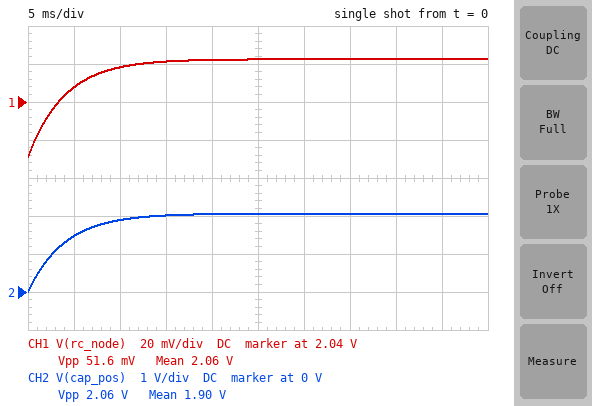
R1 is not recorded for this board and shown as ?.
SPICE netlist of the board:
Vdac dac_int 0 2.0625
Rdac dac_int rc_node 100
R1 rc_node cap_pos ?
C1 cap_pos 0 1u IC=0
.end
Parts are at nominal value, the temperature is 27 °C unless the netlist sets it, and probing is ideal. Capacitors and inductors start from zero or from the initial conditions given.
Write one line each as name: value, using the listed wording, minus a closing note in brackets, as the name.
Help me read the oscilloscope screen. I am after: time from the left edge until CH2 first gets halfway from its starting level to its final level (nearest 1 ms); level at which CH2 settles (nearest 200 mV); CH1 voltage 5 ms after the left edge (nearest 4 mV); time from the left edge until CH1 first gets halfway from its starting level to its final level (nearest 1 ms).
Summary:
time from the left edge until CH2 first gets halfway from its starting level to its final level: 3 ms
level at which CH2 settles: 2.0 V
CH1 voltage 5 ms after the left edge: 2.048 V
time from the left edge until CH1 first gets halfway from its starting level to its final level: 3 ms
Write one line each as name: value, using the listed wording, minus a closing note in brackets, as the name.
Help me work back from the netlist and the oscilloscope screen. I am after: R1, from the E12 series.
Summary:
R1, from the E12 series: 3.9 kΩ
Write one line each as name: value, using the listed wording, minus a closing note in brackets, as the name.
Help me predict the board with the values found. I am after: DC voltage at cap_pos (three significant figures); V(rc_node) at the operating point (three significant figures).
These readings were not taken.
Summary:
DC voltage at cap_pos: 2.06 V
V(rc_node) at the operating point: 2.06 V
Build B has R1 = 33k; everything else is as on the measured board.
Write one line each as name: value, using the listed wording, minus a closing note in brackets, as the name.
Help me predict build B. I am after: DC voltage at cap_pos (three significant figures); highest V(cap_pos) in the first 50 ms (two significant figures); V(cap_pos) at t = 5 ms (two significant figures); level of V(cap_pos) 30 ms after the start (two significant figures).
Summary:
DC voltage at cap_pos: 2.06 V
highest V(cap_pos) in the first 50 ms: 1.6 V
V(cap_pos) at t = 5 ms: 290 mV
level of V(cap_pos) 30 ms after the start: 1.2 V
